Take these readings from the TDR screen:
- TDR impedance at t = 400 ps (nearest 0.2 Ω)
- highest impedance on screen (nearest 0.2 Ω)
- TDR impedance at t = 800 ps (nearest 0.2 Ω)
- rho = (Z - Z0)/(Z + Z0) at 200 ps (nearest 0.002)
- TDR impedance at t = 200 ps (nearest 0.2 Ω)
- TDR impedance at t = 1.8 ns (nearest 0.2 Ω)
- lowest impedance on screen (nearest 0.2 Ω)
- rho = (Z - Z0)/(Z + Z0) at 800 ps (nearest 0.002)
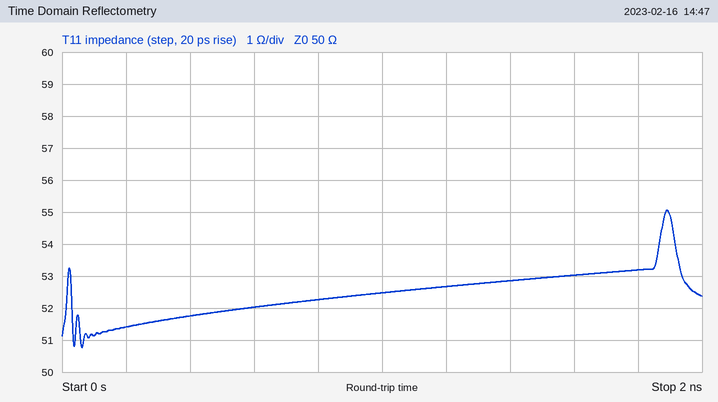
51.8 Ω
55.0 Ω
52.2 Ω
+0.014
51.4 Ω
53.2 Ω
50.8 Ω
+0.022
